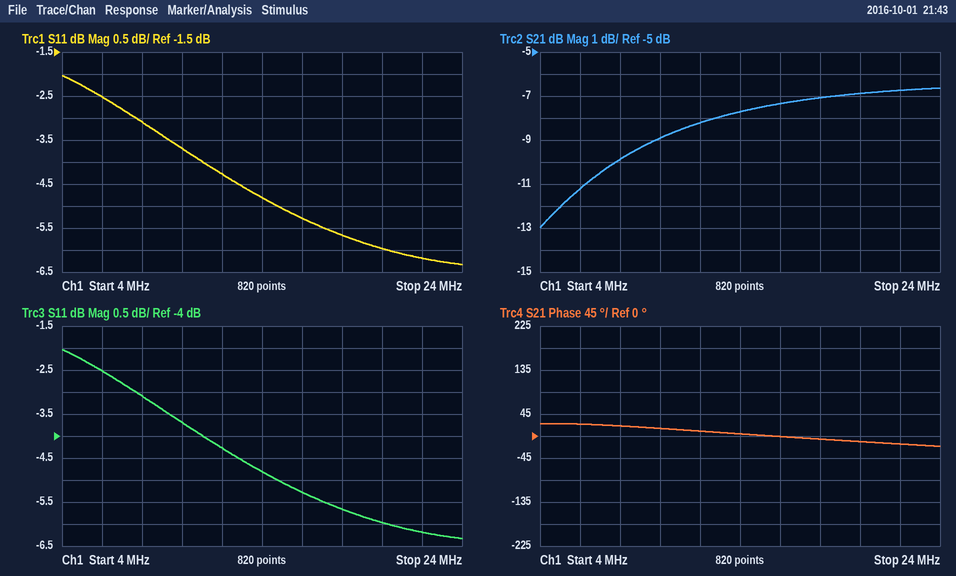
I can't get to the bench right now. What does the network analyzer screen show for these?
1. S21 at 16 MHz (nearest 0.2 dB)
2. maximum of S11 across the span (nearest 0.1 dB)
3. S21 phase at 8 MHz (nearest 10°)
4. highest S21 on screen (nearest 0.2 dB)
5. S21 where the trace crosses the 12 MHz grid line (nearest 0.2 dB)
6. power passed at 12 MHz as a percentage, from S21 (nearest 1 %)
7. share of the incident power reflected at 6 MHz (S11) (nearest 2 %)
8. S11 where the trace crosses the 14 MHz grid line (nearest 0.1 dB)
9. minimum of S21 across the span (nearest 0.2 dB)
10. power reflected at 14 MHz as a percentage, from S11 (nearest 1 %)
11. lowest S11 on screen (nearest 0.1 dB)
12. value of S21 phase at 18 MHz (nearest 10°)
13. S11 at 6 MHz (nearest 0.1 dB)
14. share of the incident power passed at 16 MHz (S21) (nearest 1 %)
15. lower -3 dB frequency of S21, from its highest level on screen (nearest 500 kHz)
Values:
-7.4 dB
-2.0 dB
20°
-6.6 dB
-8.2 dB
15 %
56 %
-4.8 dB
-13.0 dB
33 %
-6.3 dB
-10°
-2.5 dB
18 %
8.5 MHz
